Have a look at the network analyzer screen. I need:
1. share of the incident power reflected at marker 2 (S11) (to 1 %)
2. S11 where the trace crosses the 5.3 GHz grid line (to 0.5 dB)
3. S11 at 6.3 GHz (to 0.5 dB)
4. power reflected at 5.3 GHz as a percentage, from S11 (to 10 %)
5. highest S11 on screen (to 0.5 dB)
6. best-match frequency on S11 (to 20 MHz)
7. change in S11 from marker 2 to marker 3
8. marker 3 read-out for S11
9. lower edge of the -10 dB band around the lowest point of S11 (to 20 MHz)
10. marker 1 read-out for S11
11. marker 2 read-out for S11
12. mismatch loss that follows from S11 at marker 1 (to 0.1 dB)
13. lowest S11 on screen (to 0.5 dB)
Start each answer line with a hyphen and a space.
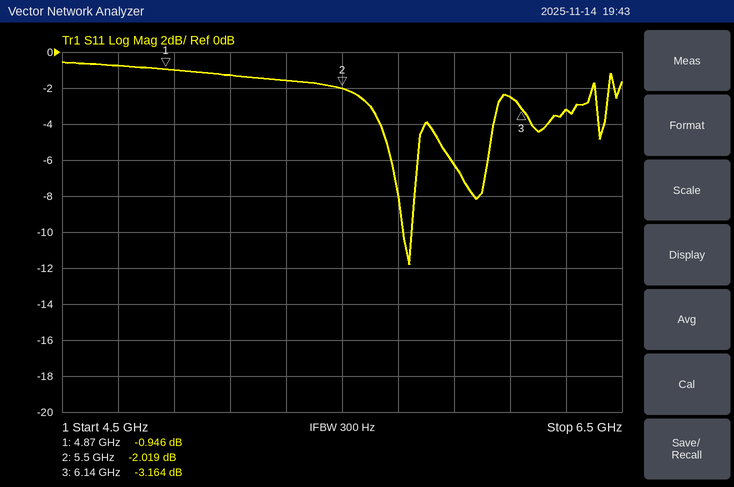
- 63 %
- -1.5 dB
- -3.0 dB
- 70 %
- -0.5 dB
- 5.74 GHz
- -1.145 dB
- -3.164 dB
- 5.72 GHz
- -0.946 dB
- -2.019 dB
- 7.1 dB
- -12.0 dB
